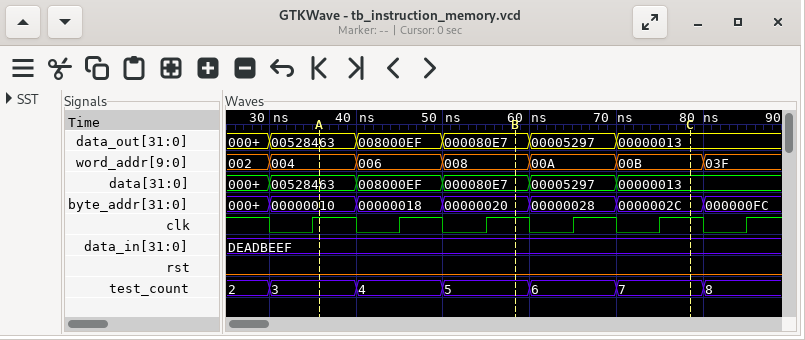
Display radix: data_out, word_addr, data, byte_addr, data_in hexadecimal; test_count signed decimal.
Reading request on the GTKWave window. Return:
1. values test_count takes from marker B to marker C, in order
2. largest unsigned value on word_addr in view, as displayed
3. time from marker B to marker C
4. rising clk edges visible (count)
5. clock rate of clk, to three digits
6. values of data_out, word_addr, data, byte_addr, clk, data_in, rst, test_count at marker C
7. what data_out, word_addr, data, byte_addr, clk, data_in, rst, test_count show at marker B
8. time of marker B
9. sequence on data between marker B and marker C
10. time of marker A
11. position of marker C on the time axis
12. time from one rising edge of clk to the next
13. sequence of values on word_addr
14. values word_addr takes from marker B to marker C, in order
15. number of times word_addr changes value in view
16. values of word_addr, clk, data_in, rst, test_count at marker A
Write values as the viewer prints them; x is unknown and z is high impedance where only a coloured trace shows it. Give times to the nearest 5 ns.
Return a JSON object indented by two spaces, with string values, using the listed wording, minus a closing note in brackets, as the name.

{
  "values test_count takes from marker B to marker C, in order": "5, 6, 7",
  "largest unsigned value on word_addr in view, as displayed": "03F",
  "time from marker B to marker C": "20 ns",
  "rising clk edges visible": "6",
  "clock rate of clk, to three digits": "100 MHz",
  "values of data_out, word_addr, data, byte_addr, clk, data_in, rst, test_count at marker C": "data_out=00000013, word_addr=00B, data=00000013, byte_addr=0000002C, clk=1, data_in=DEADBEEF, rst=0, test_count=7",
  "what data_out, word_addr, data, byte_addr, clk, data_in, rst, test_count show at marker B": "data_out=000080E7, word_addr=008, data=000080E7, byte_addr=00000020, clk=1, data_in=DEADBEEF, rst=0, test_count=5",
  "time of marker B": "60 ns",
  "sequence on data between marker B and marker C": "000080E7, 00005297, 00000013",
  "time of marker A": "35 ns",
  "position of marker C on the time axis": "80 ns",
  "time from one rising edge of clk to the next": "10 ns",
  "sequence of values on word_addr": "002, 004, 006, 008, 00A, 00B, 03F",
  "values word_addr takes from marker B to marker C, in order": "008, 00A, 00B",
  "number of times word_addr changes value in view": "6",
  "values of word_addr, clk, data_in, rst, test_count at marker A": "word_addr=004, clk=1, data_in=DEADBEEF, rst=0, test_count=3"
}
